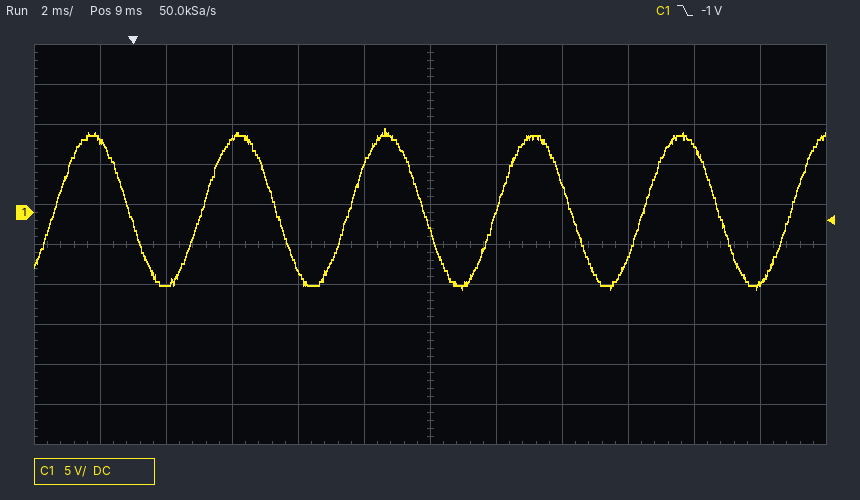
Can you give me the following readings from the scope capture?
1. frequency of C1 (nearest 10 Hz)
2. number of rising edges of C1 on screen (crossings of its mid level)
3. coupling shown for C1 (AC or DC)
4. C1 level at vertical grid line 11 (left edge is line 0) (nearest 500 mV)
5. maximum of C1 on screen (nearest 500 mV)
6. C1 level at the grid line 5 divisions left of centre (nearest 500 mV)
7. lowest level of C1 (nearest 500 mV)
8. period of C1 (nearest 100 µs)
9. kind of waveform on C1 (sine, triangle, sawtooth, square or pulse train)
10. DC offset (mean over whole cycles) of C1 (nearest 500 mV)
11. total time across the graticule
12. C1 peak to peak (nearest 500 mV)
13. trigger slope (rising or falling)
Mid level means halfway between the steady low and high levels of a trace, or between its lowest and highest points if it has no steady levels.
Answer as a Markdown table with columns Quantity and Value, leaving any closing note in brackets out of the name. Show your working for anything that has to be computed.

| Quantity | Value |
|---|---|
| frequency of C1 | 1 / 4.5 ms ≈ 222 Hz, so 220 Hz to the nearest 10 Hz |
| number of rising edges of C1 on screen | 6 |
| coupling shown for C1 | DC |
| C1 level at vertical grid line 11 (left edge is line 0) | -9.0 V |
| maximum of C1 on screen | 10.5 V |
| C1 level at the grid line 5 divisions left of centre | 9.0 V |
| lowest level of C1 | -9.5 V |
| period of C1 | 4.5 ms |
| kind of waveform on C1 | sine |
| DC offset (mean over whole cycles) of C1 | (10.5 V + (-9.5 V)) / 2 ≈ 500 mV |
| total time across the graticule | 24 ms |
| C1 peak to peak | 10.5 V − (-9.5 V) = 20.0 V |
| trigger slope | falling |
